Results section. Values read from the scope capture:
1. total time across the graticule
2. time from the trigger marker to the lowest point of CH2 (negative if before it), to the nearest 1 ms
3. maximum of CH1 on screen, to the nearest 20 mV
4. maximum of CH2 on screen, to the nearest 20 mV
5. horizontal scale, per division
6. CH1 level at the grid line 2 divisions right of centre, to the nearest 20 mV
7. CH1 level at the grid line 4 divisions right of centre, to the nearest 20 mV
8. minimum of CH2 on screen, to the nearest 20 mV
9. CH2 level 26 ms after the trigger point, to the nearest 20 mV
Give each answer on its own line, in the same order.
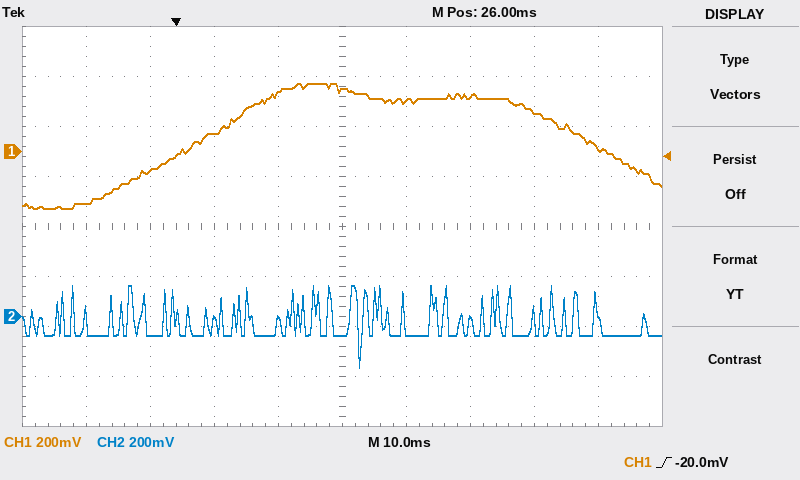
100 ms
+29 ms
280 mV
120 mV
10 ms
220 mV
20 mV
-200 mV
-80 mV
